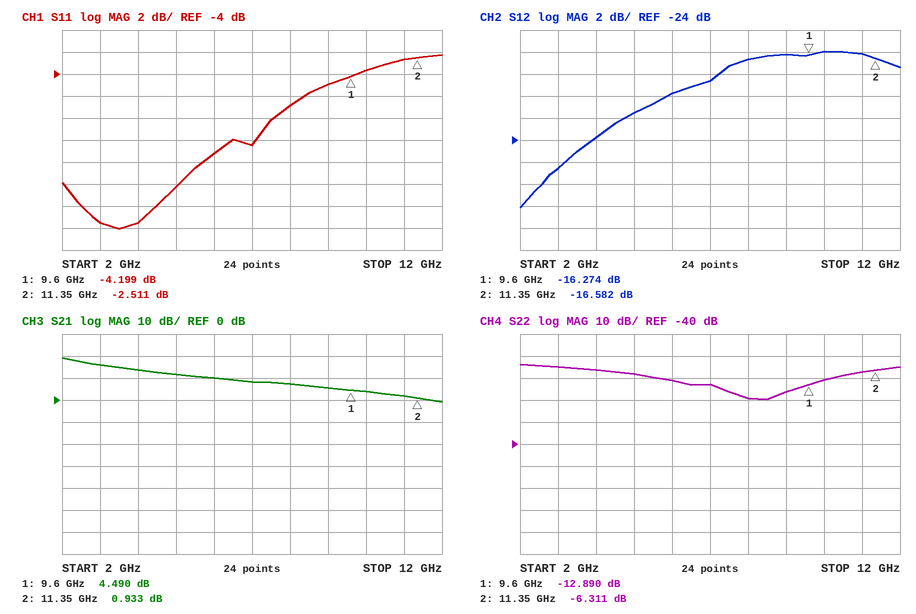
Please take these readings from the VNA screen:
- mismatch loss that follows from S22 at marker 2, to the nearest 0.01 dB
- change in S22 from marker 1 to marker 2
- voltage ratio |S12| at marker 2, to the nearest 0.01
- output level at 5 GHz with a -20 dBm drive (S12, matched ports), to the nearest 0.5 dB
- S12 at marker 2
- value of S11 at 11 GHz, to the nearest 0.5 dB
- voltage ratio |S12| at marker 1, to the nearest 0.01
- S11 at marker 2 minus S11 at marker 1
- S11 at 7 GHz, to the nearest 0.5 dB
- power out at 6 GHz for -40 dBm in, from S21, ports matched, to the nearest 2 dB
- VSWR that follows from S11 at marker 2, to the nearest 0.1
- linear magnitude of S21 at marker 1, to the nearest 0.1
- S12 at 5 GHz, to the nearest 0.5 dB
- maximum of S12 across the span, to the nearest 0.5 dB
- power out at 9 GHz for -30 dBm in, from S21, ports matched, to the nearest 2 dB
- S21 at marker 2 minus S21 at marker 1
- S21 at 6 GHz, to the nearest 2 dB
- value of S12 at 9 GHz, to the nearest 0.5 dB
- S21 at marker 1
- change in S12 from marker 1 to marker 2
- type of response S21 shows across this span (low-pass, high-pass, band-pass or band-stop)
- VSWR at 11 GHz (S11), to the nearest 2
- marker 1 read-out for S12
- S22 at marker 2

1.16 dB
6.579 dB
0.15
-41.5 dBm
-16.582 dB
-2.5 dB
0.15
1.688 dB
-10.5 dB
-30 dBm
7.0
1.7
-21.5 dB
-16.0 dB
-24 dBm
-3.557 dB
10 dB
-16.0 dB
4.490 dB
-0.308 dB
low-pass
6
-16.274 dB
-6.311 dB
